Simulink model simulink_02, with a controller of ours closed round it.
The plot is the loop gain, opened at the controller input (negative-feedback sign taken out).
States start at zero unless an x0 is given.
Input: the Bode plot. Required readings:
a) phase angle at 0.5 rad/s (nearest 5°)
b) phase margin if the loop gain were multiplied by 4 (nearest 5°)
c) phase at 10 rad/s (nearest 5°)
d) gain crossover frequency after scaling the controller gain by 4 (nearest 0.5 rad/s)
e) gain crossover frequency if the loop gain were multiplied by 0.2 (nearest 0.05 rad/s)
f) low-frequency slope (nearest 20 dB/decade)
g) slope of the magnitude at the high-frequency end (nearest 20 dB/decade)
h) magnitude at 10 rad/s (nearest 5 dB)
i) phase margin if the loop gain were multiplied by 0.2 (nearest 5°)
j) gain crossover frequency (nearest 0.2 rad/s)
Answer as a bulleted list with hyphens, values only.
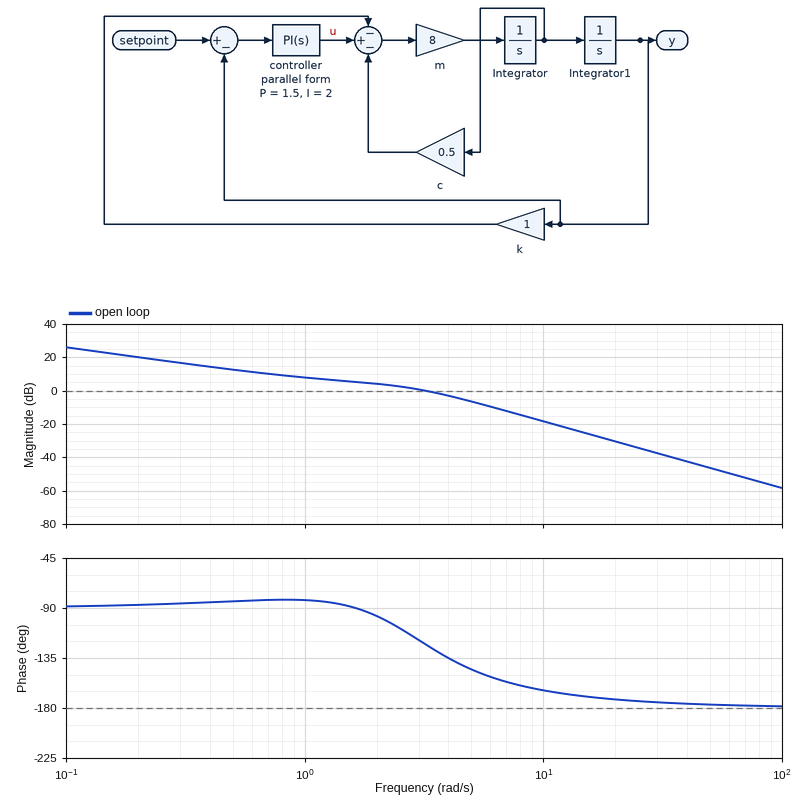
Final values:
- -85°
- 25°
- -165°
- 7.0 rad/s
- 0.40 rad/s
- -20 dB/decade
- -40 dB/decade
- -20 dB
- 95°
- 3.2 rad/s
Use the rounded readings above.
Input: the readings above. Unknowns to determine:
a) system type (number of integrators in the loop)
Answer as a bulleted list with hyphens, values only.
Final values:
- 1
